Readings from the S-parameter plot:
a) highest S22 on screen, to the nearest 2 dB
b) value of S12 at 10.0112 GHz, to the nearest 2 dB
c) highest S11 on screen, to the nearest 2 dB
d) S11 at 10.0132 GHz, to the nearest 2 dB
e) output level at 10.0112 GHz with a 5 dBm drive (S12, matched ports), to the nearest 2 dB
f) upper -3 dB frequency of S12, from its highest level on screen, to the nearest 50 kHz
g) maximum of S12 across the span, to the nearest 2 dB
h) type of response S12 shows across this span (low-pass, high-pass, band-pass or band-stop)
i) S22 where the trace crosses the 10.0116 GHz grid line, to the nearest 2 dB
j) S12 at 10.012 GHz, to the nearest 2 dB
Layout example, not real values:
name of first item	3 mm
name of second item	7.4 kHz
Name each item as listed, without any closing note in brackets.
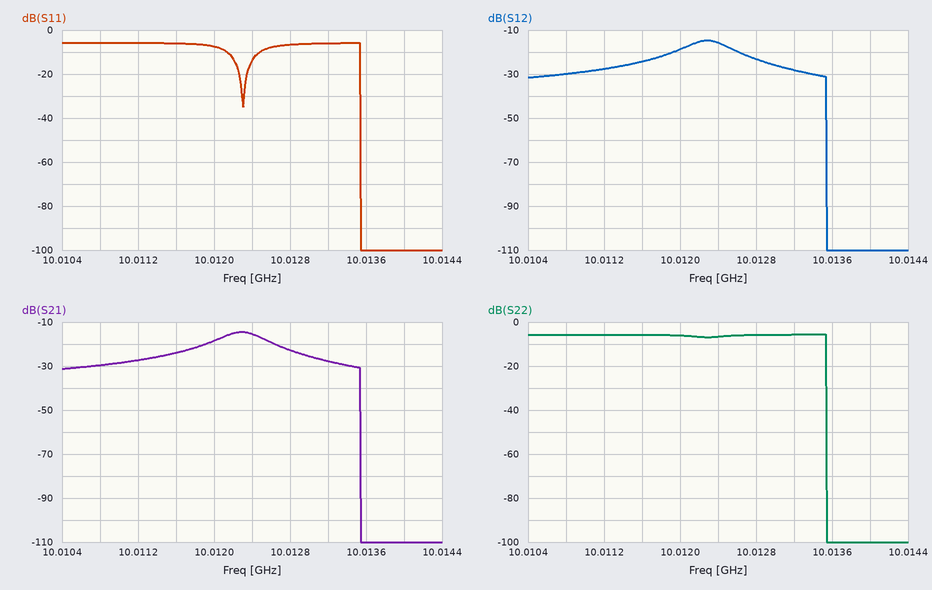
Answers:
highest S22 on screen, to the nearest 2 dB	-6 dB
value of S12 at 10.0112 GHz, to the nearest 2 dB	-28 dB
highest S11 on screen, to the nearest 2 dB	-6 dB
S11 at 10.0132 GHz, to the nearest 2 dB	-6 dB
output level at 10.0112 GHz with a 5 dBm drive (S12, matched ports), to the nearest 2 dB	-22 dBm
upper -3 dB frequency of S12, from its highest level on screen, to the nearest 50 kHz	10.01250 GHz
maximum of S12 across the span, to the nearest 2 dB	-14 dB
type of response S12 shows across this span	band-pass
S22 where the trace crosses the 10.0116 GHz grid line, to the nearest 2 dB	-6 dB
S12 at 10.012 GHz, to the nearest 2 dB	-18 dB
